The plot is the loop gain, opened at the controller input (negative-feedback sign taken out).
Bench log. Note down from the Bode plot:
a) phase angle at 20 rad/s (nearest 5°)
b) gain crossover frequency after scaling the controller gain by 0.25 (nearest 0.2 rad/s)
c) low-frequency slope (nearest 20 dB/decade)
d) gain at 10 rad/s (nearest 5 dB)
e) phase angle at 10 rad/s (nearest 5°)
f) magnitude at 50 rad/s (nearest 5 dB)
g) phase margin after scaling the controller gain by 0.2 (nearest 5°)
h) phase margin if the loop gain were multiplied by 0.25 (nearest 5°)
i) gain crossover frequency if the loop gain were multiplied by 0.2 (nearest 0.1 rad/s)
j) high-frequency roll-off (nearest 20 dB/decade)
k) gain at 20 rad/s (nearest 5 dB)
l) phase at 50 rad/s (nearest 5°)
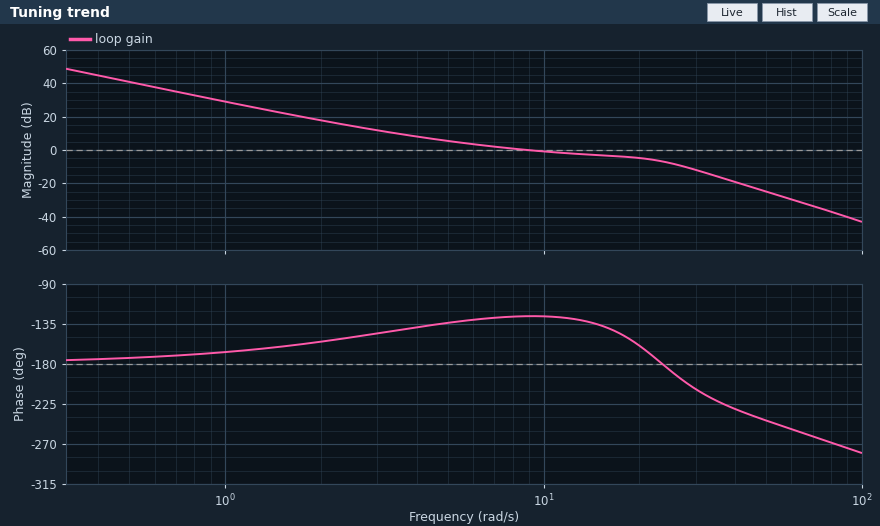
-160°
3.0 rad/s
-40 dB/decade
0 dB
-125°
-25 dB
30°
35°
2.6 rad/s
-60 dB/decade
-5 dB
-245°
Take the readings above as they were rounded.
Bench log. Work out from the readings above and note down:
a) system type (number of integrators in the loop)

2
